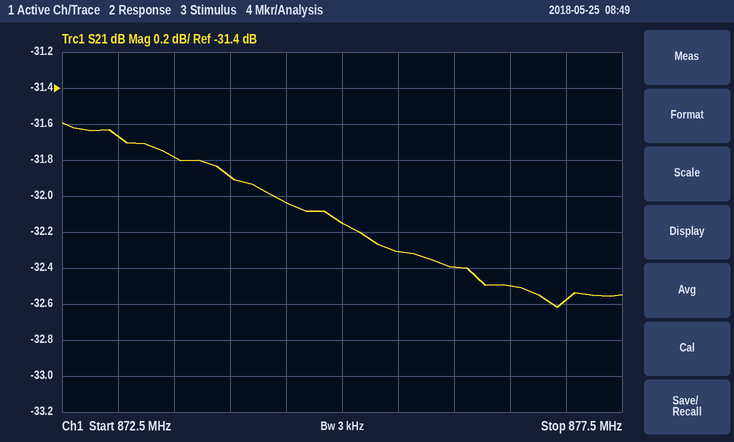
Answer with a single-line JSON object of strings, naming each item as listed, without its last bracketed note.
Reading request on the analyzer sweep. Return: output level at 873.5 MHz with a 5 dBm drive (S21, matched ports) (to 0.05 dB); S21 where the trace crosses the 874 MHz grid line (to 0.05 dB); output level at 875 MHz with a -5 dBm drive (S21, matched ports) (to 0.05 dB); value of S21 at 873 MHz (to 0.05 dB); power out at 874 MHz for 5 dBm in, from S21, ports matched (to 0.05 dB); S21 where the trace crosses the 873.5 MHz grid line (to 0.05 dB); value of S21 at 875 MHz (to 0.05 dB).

{"output level at 873.5 MHz with a 5 dBm drive (S21, matched ports)": "-26.80 dBm", "S21 where the trace crosses the 874 MHz grid line": "-31.90 dB", "output level at 875 MHz with a -5 dBm drive (S21, matched ports)": "-37.15 dBm", "value of S21 at 873 MHz": "-31.65 dB", "power out at 874 MHz for 5 dBm in, from S21, ports matched": "-26.90 dBm", "S21 where the trace crosses the 873.5 MHz grid line": "-31.80 dB", "value of S21 at 875 MHz": "-32.15 dB"}
